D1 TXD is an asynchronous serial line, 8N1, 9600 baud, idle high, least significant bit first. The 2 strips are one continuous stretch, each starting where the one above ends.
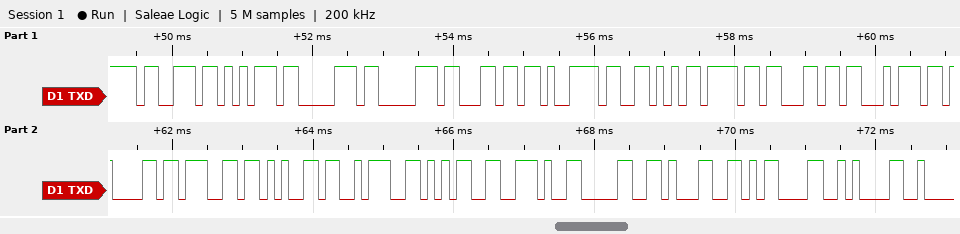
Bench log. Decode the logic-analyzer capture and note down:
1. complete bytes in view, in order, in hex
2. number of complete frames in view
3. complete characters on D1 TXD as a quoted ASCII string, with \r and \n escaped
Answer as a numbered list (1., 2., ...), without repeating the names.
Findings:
1. 73 75 70 70 6C 79 56 6F 6C 74 61 67 65 3A 35 2E 30 31 0D 0A
2. 20
3. "supplyVoltage:5.01\r\n"
